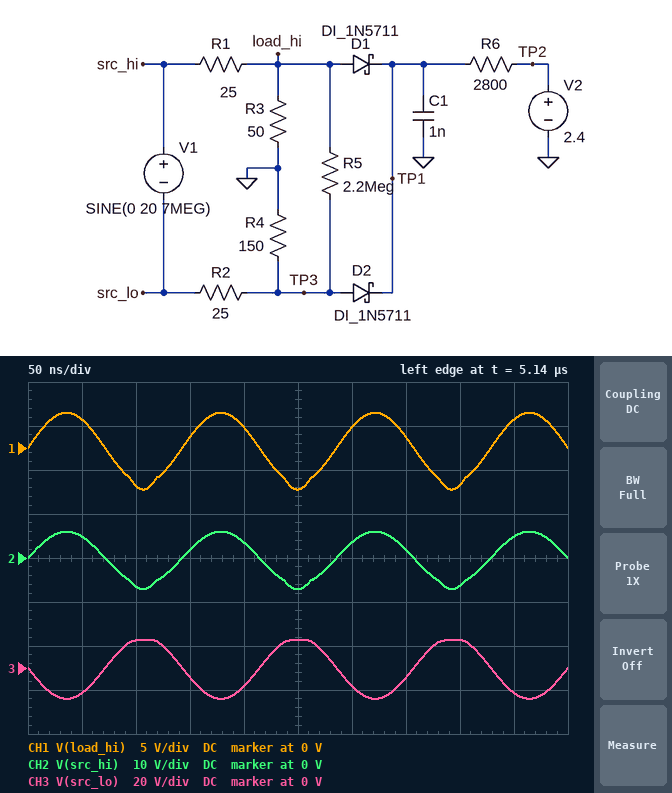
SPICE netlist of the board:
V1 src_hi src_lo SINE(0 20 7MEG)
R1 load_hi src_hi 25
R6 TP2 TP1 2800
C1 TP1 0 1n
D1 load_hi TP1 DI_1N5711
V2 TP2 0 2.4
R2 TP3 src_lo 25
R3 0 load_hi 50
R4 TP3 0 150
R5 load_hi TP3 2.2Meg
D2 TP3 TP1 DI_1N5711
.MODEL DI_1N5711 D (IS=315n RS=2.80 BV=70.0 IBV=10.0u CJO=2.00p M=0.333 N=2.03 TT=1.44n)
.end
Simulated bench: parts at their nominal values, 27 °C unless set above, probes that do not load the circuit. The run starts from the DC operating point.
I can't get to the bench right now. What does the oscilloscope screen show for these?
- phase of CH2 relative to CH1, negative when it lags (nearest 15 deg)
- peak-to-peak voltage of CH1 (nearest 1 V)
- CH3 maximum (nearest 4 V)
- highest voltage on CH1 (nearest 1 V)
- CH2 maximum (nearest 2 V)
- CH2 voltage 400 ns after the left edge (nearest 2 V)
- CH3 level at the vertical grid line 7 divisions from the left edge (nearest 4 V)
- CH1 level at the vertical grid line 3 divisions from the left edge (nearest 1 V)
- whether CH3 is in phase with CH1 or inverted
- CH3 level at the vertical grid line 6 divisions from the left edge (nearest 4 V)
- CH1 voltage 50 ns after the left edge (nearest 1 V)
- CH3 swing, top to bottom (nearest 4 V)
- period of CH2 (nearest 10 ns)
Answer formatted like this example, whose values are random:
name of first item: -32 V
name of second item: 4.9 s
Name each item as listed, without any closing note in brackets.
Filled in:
phase of CH2 relative to CH1, negative when it lags: 0 deg
peak-to-peak voltage of CH1: 9 V
CH3 maximum: 12 V
highest voltage on CH1: 4 V
CH2 maximum: 6 V
CH2 voltage 400 ns after the left edge: -6 V
CH3 level at the vertical grid line 7 divisions from the left edge: -4 V
CH1 level at the vertical grid line 3 divisions from the left edge: 1 V
whether CH3 is in phase with CH1 or inverted: inverted
CH3 level at the vertical grid line 6 divisions from the left edge: -8 V
CH1 voltage 50 ns after the left edge: 3 V
CH3 swing, top to bottom: 28 V
period of CH2: 140 ns
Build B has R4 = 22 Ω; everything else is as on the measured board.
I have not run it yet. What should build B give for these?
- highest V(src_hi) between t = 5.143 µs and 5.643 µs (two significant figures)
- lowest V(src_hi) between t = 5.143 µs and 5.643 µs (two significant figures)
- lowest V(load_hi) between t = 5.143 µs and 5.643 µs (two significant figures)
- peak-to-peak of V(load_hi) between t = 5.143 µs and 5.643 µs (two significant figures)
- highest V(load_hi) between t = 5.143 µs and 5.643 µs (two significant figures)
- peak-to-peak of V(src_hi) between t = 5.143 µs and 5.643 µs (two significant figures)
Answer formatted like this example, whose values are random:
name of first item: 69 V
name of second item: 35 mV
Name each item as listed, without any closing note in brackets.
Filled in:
highest V(src_hi) between t = 5.143 µs and 5.643 µs: 12 V
lowest V(src_hi) between t = 5.143 µs and 5.643 µs: -12 V
lowest V(load_hi) between t = 5.143 µs and 5.643 µs: -8.2 V
peak-to-peak of V(load_hi) between t = 5.143 µs and 5.643 µs: 16 V
highest V(load_hi) between t = 5.143 µs and 5.643 µs: 7.7 V
peak-to-peak of V(src_hi) between t = 5.143 µs and 5.643 µs: 24 V
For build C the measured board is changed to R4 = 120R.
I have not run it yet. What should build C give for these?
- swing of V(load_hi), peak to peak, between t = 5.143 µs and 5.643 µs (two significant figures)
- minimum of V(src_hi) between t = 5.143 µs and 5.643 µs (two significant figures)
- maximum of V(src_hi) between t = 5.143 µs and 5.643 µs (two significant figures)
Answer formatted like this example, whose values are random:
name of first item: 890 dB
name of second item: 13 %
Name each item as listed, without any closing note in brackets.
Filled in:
swing of V(load_hi), peak to peak, between t = 5.143 µs and 5.643 µs: 9.7 V
minimum of V(src_hi) between t = 5.143 µs and 5.643 µs: -7.7 V
maximum of V(src_hi) between t = 5.143 µs and 5.643 µs: 6.8 V
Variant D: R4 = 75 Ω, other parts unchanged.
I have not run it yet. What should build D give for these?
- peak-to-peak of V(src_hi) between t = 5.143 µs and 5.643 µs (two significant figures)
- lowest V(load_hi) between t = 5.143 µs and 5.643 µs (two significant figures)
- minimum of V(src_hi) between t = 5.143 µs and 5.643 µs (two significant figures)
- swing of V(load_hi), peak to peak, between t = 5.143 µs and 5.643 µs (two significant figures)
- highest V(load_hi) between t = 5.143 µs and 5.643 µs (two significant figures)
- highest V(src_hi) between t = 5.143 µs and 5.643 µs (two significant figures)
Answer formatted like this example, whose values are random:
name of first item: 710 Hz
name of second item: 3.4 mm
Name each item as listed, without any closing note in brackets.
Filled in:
peak-to-peak of V(src_hi) between t = 5.143 µs and 5.643 µs: 18 V
lowest V(load_hi) between t = 5.143 µs and 5.643 µs: -6.1 V
minimum of V(src_hi) between t = 5.143 µs and 5.643 µs: -9.1 V
swing of V(load_hi), peak to peak, between t = 5.143 µs and 5.643 µs: 12 V
highest V(load_hi) between t = 5.143 µs and 5.643 µs: 5.7 V
highest V(src_hi) between t = 5.143 µs and 5.643 µs: 8.6 V
